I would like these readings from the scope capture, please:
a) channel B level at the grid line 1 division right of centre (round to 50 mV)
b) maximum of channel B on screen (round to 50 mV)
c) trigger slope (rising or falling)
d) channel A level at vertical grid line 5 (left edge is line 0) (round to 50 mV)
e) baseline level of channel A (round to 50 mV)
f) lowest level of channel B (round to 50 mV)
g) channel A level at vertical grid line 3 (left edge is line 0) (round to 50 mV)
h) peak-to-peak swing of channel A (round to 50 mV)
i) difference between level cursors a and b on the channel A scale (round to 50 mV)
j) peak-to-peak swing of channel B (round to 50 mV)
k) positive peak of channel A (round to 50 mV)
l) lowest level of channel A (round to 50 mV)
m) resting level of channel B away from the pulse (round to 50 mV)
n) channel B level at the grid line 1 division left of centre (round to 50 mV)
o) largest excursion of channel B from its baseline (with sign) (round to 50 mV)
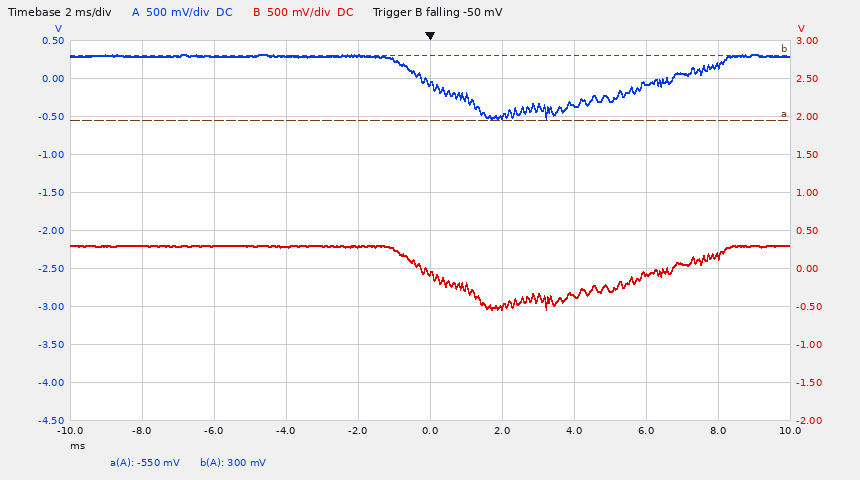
-500 mV
300 mV
falling
-50 mV
300 mV
-550 mV
300 mV
850 mV
850 mV
850 mV
300 mV
-550 mV
300 mV
300 mV
-850 mV
